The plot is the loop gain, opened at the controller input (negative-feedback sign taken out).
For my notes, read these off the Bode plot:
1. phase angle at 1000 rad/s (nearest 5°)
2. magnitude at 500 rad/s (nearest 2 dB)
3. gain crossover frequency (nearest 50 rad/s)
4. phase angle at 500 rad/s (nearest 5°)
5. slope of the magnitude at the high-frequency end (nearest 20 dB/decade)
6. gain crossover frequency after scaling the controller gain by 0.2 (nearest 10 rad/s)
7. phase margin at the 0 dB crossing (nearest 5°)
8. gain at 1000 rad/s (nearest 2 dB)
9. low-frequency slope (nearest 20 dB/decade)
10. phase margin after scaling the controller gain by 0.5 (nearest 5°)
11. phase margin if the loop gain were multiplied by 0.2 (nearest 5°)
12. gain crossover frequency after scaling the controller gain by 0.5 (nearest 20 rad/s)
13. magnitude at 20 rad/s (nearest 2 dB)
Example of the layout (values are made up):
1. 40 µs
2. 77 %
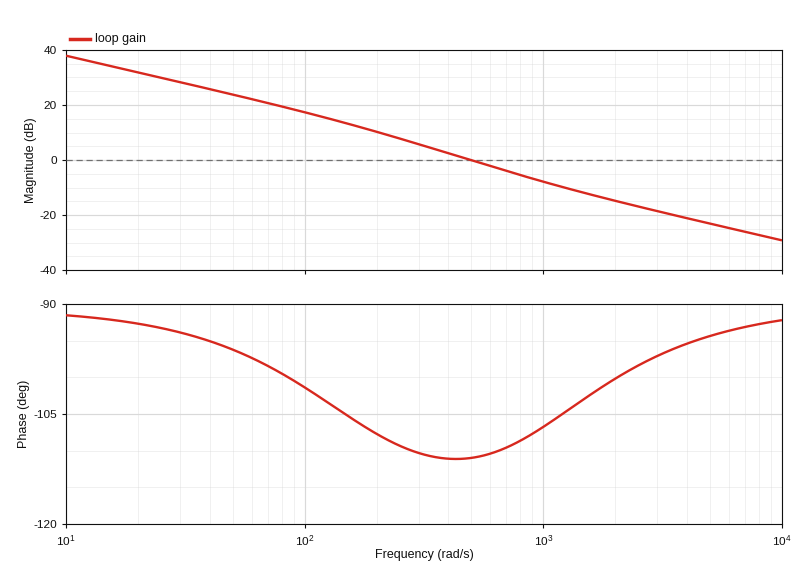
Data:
1. -105°
2. 0 dB
3. 500 rad/s
4. -110°
5. -20 dB/decade
6. 140 rad/s
7. 70°
8. -8 dB
9. -20 dB/decade
10. 70°
11. 75°
12. 300 rad/s
13. 32 dB
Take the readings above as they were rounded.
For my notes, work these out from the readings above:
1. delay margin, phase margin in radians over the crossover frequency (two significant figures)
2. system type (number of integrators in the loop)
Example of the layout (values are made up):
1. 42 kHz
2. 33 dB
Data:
1. 0.0024 s
2. 1
